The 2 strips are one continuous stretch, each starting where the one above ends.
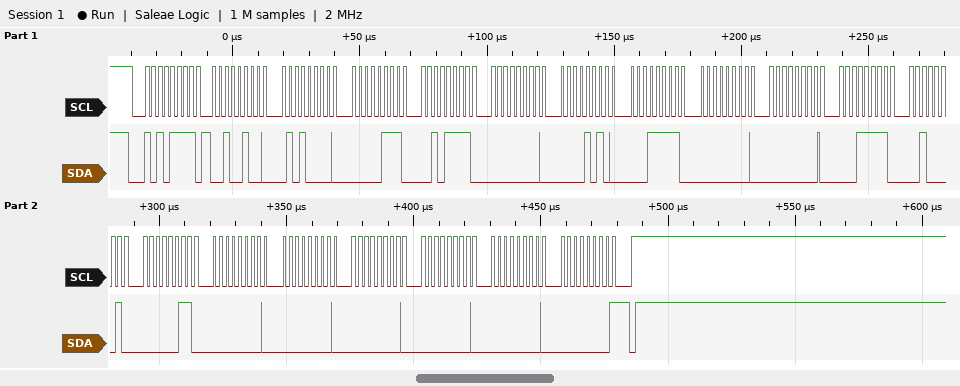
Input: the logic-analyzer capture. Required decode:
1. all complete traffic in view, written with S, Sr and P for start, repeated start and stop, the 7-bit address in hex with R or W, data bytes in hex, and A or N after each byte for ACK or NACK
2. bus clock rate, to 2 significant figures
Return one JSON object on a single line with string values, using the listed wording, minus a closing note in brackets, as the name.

{"all complete traffic in view, written with S, Sr and P for start, repeated start and stop, the 7-bit address in hex with R or W, data bytes in hex, and A or N after each byte for ACK or NACK": "S 57R A 24 A 50 A 07 A 2F A 00 A 0A A 1F A 00 A 00 A 1F A 21 A 03 A 00 A 00 A 00 A 00 A 00 A 00 N P", "bus clock rate, to 2 significant figures": "400 kHz"}
